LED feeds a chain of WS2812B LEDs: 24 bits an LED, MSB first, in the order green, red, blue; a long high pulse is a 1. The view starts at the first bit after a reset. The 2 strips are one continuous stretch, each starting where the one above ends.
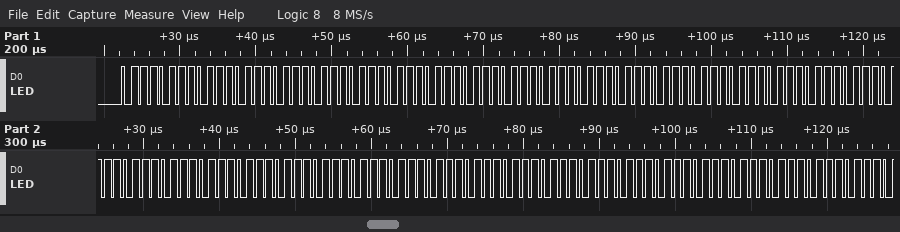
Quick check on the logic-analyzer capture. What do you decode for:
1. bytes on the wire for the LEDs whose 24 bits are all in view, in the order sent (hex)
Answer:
77 77 77 77 77 77 77 77 77 77 77 77 77 77 77 77 77 77
